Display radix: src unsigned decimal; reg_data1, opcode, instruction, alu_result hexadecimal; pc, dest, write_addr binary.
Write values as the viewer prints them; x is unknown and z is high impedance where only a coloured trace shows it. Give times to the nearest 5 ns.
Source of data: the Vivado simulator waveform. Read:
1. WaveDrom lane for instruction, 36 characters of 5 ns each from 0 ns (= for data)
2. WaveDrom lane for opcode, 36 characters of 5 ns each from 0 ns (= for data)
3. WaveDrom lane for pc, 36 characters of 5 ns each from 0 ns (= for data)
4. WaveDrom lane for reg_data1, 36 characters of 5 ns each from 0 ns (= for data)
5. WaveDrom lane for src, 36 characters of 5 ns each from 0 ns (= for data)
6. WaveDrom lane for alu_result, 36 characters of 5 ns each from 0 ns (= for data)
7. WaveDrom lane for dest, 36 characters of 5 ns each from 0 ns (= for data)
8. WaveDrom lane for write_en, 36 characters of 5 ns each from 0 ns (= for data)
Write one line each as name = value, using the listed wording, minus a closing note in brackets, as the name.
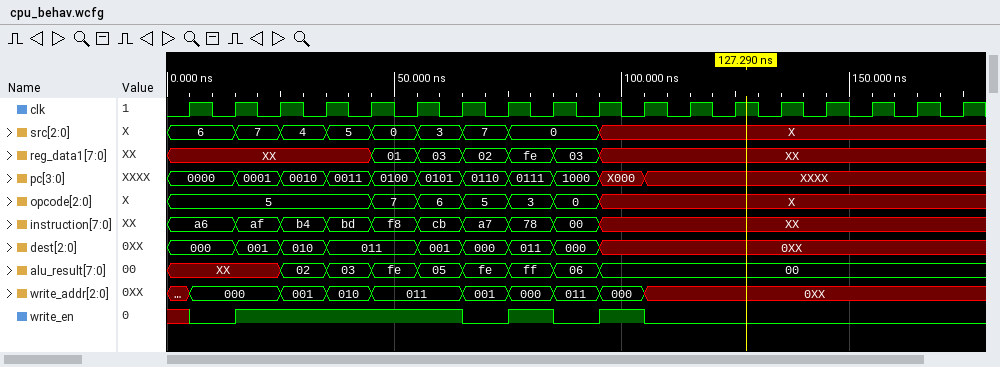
WaveDrom lane for instruction, 36 characters of 5 ns each from 0 ns = {name: 'instruction', wave: '=..=.=.=.=.=.=.=.=.x................', data: 'a6 af b4 bd f8 cb a7 78 00'}
WaveDrom lane for opcode, 36 characters of 5 ns each from 0 ns = {name: 'opcode', wave: '=........=.=.=.=.=.x................', data: '5 7 6 5 3 0'}
WaveDrom lane for pc, 36 characters of 5 ns each from 0 ns = {name: 'pc', wave: '=..=.=.=.=.=.=.=.=.=.x..............', data: '0000 0001 0010 0011 0100 0101 0110 0111 1000 X000'}
WaveDrom lane for reg_data1, 36 characters of 5 ns each from 0 ns = {name: 'reg_data1', wave: 'x........=.=.=.=.=.x................', data: '01 03 02 fe 03'}
WaveDrom lane for src, 36 characters of 5 ns each from 0 ns = {name: 'src', wave: '=..=.=.=.=.=.=.=...x................', data: '6 7 4 5 0 3 7 0'}
WaveDrom lane for alu_result, 36 characters of 5 ns each from 0 ns = {name: 'alu_result', wave: 'x....=.=.=.=.=.=.=.=................', data: '02 03 fe 05 fe ff 06 00'}
WaveDrom lane for dest, 36 characters of 5 ns each from 0 ns = {name: 'dest', wave: '=..=.=.=...=.=.=.=.=................', data: '000 001 010 011 001 000 011 000 0XX'}
WaveDrom lane for write_en, 36 characters of 5 ns each from 0 ns = {name: 'write_en', wave: 'x0.1.........0.1.0.1.0..............'}
